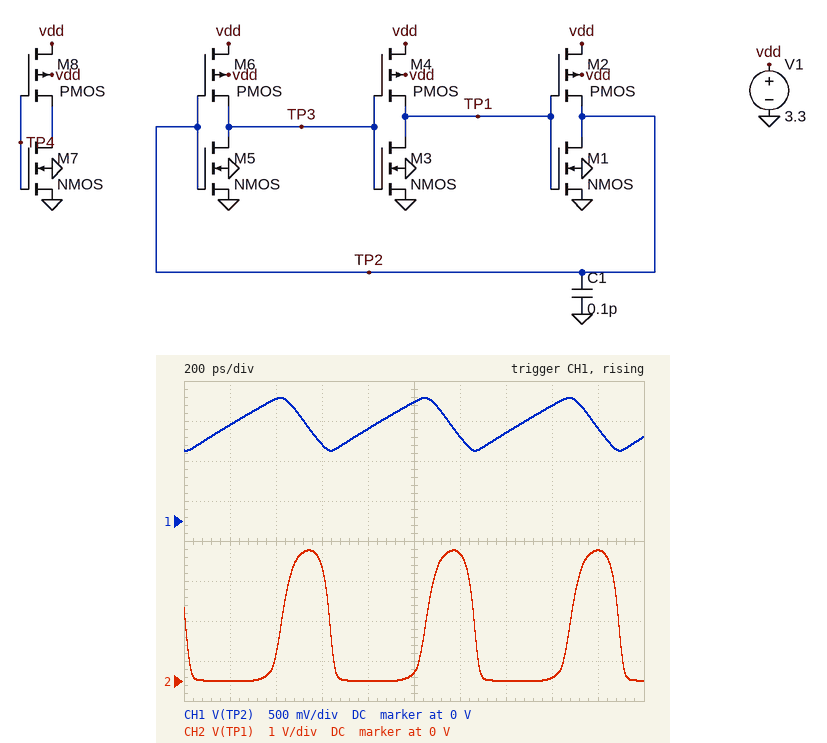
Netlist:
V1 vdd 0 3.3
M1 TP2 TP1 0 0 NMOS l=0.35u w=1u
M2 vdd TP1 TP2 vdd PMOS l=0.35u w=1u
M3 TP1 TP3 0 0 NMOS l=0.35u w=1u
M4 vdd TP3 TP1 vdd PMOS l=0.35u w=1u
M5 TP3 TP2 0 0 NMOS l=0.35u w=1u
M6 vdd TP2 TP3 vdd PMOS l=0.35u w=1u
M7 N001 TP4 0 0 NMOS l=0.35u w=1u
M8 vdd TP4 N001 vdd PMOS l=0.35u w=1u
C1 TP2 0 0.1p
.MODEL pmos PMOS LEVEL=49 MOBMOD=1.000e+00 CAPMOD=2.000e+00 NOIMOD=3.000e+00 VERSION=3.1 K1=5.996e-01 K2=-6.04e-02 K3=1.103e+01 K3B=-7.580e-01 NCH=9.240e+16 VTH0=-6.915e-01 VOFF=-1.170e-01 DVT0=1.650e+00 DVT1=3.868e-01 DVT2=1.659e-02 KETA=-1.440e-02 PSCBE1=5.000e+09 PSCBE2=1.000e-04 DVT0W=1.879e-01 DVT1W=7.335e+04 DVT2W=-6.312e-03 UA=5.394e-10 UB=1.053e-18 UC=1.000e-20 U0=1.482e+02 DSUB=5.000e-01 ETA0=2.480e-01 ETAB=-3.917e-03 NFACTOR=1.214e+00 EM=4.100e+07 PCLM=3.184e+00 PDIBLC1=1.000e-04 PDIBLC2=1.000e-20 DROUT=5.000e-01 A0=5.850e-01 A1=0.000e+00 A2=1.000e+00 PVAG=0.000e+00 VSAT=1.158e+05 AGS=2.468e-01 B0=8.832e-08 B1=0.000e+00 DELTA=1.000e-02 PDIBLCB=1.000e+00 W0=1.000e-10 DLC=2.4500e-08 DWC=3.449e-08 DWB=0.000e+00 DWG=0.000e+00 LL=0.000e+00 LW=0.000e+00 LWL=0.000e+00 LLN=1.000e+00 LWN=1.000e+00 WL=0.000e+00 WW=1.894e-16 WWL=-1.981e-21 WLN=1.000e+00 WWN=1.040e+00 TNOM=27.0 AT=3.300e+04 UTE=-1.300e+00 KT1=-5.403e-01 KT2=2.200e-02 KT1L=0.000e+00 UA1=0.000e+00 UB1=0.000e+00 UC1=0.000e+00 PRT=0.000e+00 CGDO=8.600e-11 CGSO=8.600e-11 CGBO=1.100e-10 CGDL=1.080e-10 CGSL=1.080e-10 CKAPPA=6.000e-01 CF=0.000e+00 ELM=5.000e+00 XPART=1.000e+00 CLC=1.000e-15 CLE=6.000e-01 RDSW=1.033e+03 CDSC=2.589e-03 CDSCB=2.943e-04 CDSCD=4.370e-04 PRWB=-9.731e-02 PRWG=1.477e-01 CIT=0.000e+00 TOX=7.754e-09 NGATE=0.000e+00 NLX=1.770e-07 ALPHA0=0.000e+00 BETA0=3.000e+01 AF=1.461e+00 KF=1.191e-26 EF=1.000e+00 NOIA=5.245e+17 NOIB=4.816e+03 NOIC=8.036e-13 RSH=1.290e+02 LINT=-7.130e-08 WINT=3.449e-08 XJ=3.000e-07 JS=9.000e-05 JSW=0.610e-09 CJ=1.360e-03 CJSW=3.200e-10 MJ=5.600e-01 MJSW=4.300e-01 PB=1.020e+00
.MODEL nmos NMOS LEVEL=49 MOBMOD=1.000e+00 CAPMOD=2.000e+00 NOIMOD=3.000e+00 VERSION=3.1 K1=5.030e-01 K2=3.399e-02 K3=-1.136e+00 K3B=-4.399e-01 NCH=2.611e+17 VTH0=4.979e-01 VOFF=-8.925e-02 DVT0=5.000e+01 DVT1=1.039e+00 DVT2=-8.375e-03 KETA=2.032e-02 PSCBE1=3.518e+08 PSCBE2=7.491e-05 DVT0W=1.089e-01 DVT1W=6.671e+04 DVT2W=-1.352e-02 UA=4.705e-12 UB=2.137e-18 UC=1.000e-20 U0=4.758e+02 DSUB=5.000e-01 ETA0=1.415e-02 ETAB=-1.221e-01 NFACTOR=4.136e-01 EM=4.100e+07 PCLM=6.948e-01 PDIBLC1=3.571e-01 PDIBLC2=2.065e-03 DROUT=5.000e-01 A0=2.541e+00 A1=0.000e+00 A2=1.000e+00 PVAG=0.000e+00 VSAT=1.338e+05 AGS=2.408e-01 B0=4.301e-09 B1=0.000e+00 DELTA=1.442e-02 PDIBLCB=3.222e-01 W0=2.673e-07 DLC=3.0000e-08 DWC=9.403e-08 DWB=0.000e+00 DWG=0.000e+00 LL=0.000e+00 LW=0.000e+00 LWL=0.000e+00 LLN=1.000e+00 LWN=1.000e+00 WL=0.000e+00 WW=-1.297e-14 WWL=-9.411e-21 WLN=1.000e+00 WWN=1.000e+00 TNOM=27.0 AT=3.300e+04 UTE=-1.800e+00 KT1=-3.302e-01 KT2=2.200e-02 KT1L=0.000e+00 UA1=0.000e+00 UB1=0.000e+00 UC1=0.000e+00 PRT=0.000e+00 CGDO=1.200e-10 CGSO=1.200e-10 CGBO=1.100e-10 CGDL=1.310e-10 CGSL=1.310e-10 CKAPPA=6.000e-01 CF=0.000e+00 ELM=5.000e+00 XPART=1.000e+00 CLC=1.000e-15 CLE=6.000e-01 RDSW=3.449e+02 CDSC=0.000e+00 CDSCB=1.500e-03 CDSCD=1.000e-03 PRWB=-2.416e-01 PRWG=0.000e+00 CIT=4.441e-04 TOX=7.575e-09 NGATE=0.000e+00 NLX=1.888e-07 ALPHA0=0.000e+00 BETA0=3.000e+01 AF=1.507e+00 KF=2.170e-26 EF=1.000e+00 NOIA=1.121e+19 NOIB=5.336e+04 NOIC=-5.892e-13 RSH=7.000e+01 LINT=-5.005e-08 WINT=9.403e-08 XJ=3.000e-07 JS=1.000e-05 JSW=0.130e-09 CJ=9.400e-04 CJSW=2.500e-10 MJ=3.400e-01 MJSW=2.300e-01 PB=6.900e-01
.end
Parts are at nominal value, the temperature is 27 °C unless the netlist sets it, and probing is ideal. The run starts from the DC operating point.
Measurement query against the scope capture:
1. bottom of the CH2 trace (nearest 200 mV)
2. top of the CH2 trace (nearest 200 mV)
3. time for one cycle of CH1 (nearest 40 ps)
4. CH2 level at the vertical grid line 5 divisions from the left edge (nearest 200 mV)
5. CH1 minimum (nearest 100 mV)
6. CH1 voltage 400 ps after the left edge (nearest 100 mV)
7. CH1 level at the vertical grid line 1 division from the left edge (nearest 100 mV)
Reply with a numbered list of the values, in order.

1. 0 V
2. 3.2 V
3. 640 ps
4. 200 mV
5. 900 mV
6. 1.5 V
7. 1.2 V
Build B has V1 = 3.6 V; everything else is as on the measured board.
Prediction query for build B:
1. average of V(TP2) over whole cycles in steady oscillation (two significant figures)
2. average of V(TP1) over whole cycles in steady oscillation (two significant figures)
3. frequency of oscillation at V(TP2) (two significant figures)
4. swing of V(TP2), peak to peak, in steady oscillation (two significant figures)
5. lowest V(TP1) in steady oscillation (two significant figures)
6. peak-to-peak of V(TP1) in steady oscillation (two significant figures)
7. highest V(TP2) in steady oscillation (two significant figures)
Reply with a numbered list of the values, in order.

1. 1.3 V
2. 1.1 V
3. 1.7 GHz
4. 700 mV
5. -3.7 mV
6. 3.5 V
7. 1.7 V
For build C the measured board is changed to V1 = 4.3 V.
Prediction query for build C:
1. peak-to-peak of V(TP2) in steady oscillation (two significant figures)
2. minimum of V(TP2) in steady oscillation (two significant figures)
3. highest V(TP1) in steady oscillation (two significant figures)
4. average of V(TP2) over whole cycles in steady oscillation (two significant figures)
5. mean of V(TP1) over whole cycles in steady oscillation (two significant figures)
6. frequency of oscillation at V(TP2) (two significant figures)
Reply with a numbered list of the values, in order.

1. 780 mV
2. 1.2 V
3. 4.1 V
4. 1.6 V
5. 1.4 V
6. 2.0 GHz
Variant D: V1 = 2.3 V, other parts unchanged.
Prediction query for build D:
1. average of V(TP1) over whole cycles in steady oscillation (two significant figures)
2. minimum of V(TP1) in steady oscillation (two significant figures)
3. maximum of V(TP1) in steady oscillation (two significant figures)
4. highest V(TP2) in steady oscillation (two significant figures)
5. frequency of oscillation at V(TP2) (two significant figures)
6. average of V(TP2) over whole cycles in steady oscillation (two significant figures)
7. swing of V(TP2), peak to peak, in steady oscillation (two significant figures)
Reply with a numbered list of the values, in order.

1. 680 mV
2. -12 mV
3. 2.3 V
4. 1.1 V
5. 1.0 GHz
6. 860 mV
7. 530 mV
